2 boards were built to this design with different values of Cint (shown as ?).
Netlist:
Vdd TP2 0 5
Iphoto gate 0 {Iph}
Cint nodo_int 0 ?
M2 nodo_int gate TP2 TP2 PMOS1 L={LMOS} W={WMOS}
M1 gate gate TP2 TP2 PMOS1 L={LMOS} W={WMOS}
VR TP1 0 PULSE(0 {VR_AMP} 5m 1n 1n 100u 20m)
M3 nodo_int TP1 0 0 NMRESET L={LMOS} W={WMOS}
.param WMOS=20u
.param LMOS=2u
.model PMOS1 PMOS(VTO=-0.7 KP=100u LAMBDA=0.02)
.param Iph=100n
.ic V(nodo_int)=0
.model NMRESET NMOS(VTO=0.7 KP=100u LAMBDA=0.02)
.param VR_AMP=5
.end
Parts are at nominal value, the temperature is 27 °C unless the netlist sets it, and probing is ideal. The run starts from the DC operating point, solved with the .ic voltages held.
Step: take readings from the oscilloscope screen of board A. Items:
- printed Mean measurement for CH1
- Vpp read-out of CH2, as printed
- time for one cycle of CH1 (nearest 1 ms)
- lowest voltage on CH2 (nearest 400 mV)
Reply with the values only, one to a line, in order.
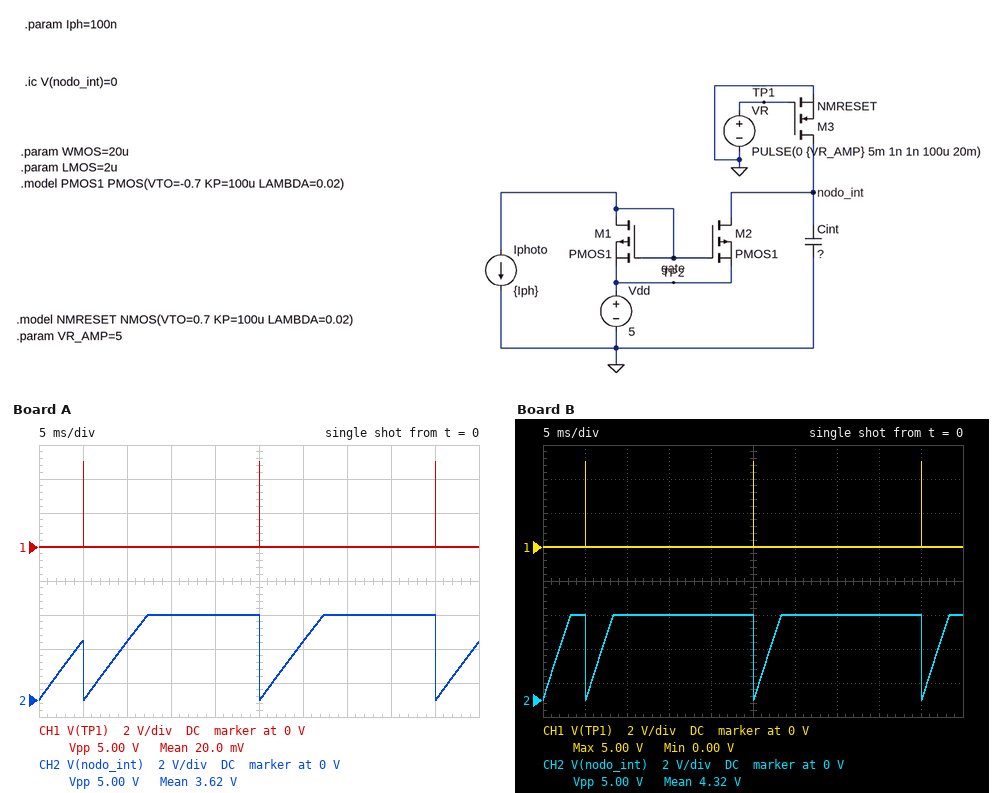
20.0 mV
5.00 V
20 ms
0 V
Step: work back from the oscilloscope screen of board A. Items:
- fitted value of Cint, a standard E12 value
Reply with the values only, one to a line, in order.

150 pF
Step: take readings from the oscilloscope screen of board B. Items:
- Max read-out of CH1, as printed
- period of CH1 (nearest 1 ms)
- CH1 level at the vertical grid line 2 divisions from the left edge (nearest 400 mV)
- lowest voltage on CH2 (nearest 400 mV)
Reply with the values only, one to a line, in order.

5.00 V
20 ms
0 V
0 V
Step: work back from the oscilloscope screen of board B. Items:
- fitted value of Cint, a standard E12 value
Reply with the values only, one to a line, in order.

68 pF
